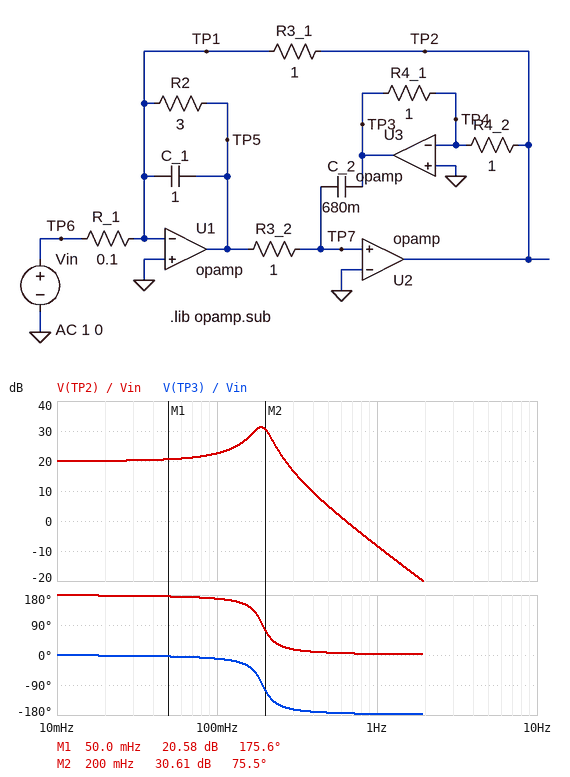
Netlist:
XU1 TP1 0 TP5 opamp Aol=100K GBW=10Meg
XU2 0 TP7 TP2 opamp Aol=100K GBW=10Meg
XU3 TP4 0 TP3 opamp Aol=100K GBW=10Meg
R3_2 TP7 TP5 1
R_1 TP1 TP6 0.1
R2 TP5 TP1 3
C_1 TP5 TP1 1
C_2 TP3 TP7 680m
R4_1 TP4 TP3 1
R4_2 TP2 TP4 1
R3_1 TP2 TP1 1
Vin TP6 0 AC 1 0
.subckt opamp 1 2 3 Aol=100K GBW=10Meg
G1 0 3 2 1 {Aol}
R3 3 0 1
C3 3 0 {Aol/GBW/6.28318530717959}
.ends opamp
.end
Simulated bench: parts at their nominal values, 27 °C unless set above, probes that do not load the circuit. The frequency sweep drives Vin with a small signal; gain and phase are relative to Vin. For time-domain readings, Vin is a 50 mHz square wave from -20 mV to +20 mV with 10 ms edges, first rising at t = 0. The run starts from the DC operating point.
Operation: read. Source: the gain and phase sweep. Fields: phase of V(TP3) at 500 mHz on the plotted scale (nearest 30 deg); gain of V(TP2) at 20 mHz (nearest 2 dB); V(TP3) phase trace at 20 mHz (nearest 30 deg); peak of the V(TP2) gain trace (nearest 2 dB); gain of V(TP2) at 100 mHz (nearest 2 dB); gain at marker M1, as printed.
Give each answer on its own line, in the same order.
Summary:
-180 deg
20 dB
0 deg
32 dB
22 dB
20.58 dB
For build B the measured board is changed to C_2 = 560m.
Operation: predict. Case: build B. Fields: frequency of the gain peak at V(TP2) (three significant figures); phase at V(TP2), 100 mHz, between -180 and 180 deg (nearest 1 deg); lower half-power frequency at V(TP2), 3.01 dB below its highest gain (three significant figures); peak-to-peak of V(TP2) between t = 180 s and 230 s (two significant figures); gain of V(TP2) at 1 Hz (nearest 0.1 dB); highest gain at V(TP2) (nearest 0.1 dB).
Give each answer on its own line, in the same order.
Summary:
209 mHz
171 deg
181 mHz
860 mV
-6.5 dB
32.1 dB
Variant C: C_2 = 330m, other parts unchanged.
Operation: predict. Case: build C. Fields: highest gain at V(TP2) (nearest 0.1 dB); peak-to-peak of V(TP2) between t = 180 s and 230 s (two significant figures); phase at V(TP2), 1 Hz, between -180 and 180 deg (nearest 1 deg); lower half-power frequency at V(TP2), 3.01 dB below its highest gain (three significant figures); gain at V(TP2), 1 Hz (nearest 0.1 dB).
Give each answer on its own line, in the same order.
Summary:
34.4 dB
990 mV
3 deg
246 mHz
-1.6 dB
